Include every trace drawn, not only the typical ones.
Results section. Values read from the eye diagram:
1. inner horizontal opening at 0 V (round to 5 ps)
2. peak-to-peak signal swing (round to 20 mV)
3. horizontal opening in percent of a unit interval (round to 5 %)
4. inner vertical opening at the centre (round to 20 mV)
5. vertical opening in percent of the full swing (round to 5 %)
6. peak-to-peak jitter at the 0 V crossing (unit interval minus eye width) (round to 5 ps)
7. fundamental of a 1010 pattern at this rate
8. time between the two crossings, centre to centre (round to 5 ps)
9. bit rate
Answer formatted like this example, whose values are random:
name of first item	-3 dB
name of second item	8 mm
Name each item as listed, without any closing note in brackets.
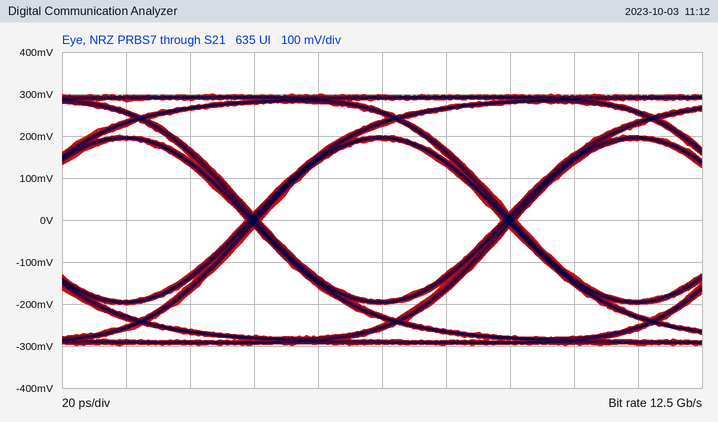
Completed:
inner horizontal opening at 0 V	75 ps
peak-to-peak signal swing	600 mV
horizontal opening in percent of a unit interval	95 %
inner vertical opening at the centre	380 mV
vertical opening in percent of the full swing	65 %
peak-to-peak jitter at the 0 V crossing (unit interval minus eye width)	5 ps
fundamental of a 1010 pattern at this rate	6.25 GHz
time between the two crossings, centre to centre	80 ps
bit rate	12.5 Gb/s
